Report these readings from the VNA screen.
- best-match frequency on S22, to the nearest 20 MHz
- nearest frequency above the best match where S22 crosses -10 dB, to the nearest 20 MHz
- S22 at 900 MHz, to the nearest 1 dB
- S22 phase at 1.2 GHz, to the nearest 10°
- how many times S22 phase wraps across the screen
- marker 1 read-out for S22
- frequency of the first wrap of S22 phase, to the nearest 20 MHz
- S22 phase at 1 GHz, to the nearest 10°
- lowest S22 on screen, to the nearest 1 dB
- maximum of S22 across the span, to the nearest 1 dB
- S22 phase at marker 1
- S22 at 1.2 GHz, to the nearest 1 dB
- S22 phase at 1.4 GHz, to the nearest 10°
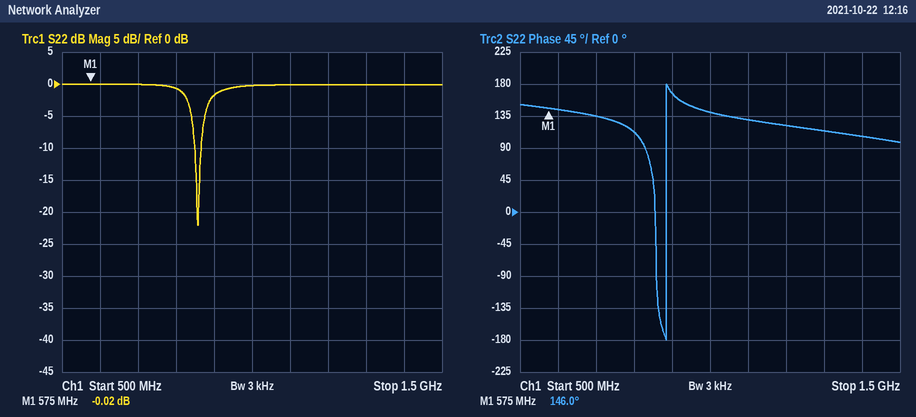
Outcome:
860 MHz
860 MHz
-2 dB
120°
1
-0.02 dB
880 MHz
140°
-22 dB
0 dB
146.0°
0 dB
110°
